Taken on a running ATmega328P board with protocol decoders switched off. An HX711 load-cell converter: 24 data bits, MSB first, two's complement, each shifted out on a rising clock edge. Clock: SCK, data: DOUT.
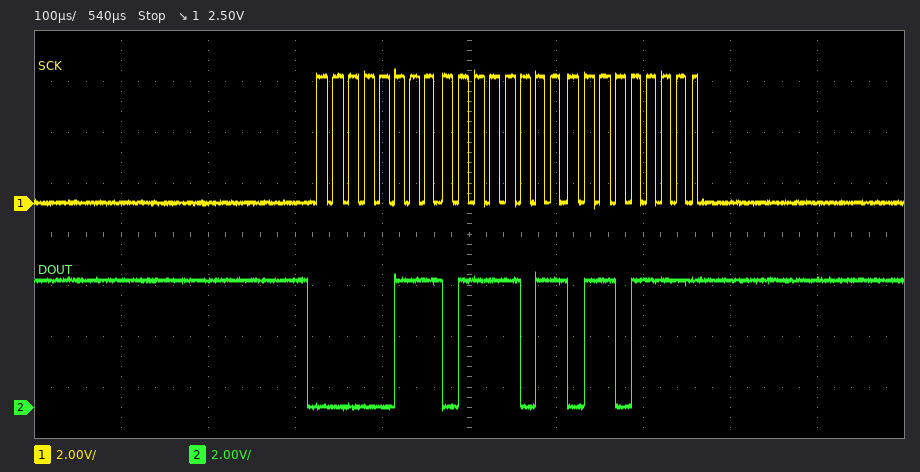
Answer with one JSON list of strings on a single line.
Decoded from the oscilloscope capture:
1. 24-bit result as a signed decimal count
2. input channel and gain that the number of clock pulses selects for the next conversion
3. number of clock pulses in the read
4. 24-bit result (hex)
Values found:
["490351", "channel A, gain 128", "25", "0x077B6F"]
